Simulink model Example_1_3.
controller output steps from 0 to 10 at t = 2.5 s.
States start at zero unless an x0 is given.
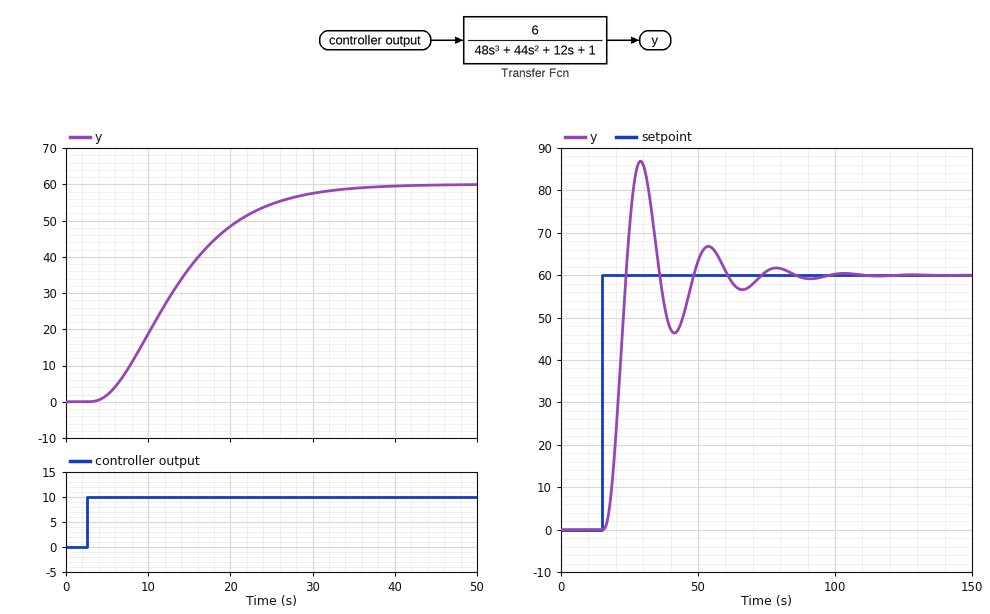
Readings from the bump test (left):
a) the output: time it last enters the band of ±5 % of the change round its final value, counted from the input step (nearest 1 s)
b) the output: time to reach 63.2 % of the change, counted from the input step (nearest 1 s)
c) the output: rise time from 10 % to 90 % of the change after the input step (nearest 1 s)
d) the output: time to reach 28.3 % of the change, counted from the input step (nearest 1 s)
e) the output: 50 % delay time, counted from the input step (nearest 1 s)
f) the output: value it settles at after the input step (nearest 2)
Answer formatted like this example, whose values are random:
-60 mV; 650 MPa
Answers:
26 s; 13 s; 18 s; 7 s; 10 s; 60
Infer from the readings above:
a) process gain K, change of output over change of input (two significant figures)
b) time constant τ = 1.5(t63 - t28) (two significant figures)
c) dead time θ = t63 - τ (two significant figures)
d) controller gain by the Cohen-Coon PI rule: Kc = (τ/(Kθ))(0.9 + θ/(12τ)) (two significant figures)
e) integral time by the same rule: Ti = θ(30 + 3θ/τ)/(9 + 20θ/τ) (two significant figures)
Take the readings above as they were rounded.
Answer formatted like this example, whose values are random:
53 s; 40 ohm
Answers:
6.0; 9.0 s; 4.0 s; 0.35; 7.0 s
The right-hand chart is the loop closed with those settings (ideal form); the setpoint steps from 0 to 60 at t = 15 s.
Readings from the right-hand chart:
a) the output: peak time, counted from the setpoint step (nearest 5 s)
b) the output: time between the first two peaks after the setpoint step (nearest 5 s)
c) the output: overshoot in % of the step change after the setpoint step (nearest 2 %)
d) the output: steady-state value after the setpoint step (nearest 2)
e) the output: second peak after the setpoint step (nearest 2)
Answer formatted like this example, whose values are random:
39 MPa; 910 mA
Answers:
15 s; 25 s; 44 %; 60; 66
